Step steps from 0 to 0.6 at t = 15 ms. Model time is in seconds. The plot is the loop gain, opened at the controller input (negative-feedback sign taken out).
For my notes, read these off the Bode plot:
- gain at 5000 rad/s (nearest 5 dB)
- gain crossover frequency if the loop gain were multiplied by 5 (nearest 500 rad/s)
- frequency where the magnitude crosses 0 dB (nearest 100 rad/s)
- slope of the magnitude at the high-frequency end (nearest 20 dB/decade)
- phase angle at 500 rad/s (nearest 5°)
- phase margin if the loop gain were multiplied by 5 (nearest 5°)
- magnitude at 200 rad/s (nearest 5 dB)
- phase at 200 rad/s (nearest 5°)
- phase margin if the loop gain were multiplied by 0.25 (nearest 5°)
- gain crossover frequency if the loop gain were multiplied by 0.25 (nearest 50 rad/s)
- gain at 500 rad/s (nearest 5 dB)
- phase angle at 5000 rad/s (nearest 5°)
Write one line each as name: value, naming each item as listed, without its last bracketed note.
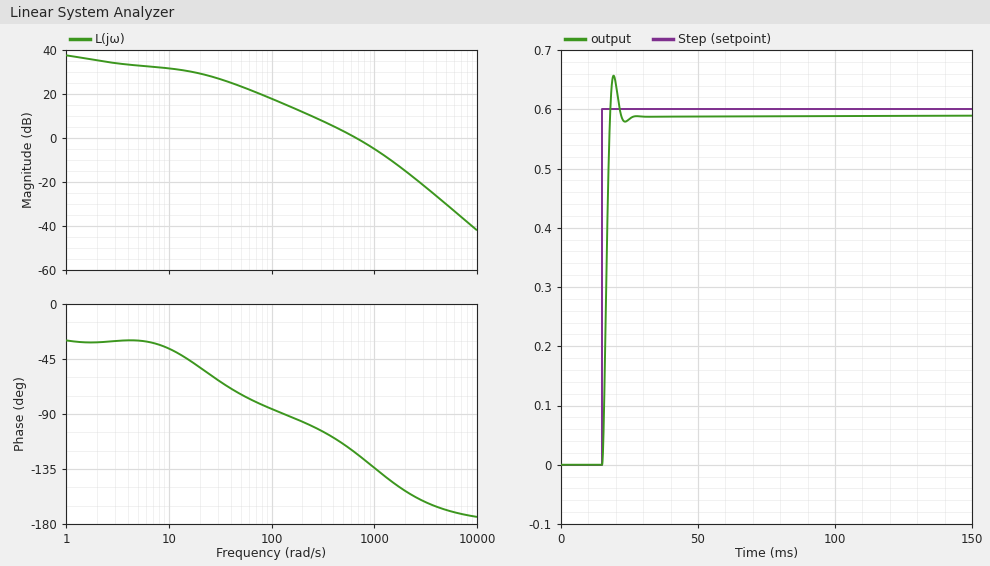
gain at 5000 rad/s: -30 dB
gain crossover frequency if the loop gain were multiplied by 5: 2000 rad/s
frequency where the magnitude crosses 0 dB: 700 rad/s
slope of the magnitude at the high-frequency end: -40 dB/decade
phase angle at 500 rad/s: -115°
phase margin if the loop gain were multiplied by 5: 30°
magnitude at 200 rad/s: 10 dB
phase at 200 rad/s: -95°
phase margin if the loop gain were multiplied by 0.25: 85°
gain crossover frequency if the loop gain were multiplied by 0.25: 200 rad/s
gain at 500 rad/s: 5 dB
phase angle at 5000 rad/s: -170°
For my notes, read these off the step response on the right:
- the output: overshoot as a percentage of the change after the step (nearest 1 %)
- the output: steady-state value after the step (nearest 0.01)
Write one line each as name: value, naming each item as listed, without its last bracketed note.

the output: overshoot as a percentage of the change after the step: 11 %
the output: steady-state value after the step: 0.59
